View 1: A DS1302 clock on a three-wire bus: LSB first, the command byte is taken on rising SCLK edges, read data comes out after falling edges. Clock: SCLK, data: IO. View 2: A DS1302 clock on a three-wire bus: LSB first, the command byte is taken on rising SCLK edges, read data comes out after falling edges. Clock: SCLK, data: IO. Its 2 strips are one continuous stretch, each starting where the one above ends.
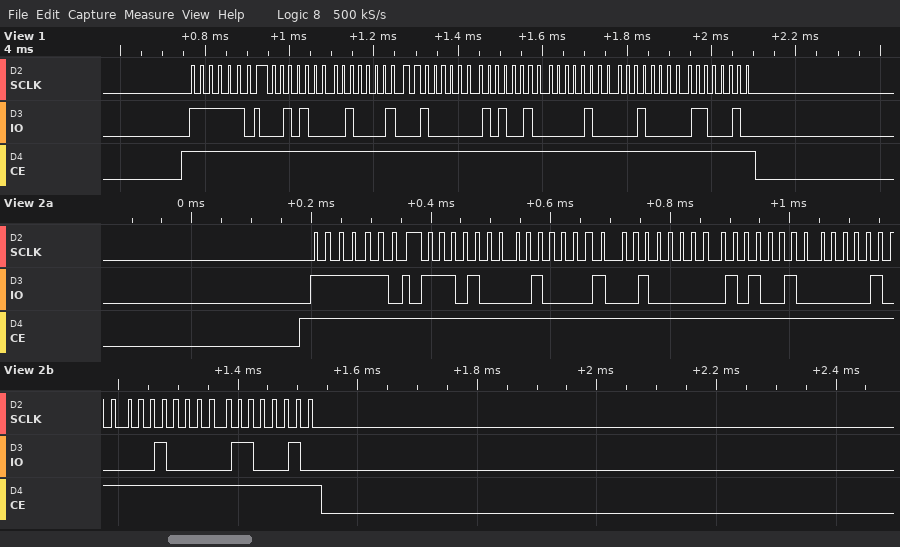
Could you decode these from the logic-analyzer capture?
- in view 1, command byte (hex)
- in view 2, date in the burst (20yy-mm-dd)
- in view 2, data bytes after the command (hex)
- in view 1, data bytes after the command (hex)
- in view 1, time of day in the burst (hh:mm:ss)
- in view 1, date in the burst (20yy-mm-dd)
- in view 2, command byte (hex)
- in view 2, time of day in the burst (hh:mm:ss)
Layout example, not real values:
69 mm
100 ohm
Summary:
0xBF
2023-10-25
17 42 02 25 10 04 23
14 42 02 25 10 04 23
02:42:14
2023-10-25
0xBF
02:42:17
